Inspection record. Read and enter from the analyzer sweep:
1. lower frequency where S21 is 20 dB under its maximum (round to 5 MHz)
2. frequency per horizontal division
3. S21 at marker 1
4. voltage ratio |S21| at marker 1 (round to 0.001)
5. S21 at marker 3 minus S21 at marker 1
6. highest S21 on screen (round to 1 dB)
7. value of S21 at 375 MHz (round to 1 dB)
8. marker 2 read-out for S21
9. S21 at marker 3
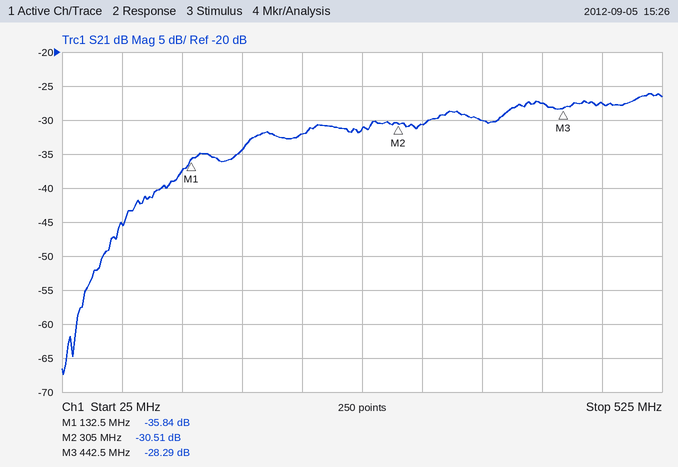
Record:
70 MHz
50 MHz
-35.84 dB
0.016
7.55 dB
-26 dB
-30 dB
-30.51 dB
-28.29 dB
